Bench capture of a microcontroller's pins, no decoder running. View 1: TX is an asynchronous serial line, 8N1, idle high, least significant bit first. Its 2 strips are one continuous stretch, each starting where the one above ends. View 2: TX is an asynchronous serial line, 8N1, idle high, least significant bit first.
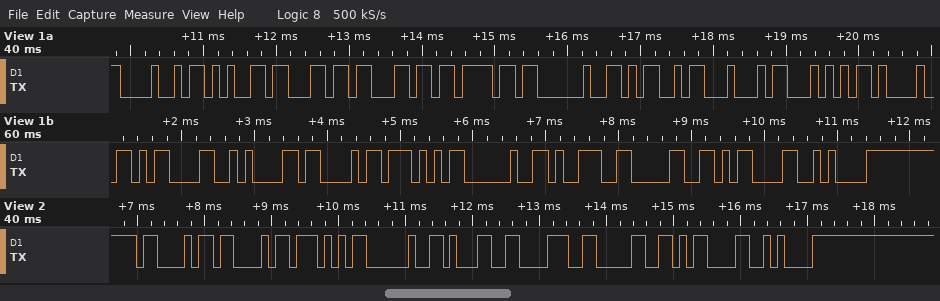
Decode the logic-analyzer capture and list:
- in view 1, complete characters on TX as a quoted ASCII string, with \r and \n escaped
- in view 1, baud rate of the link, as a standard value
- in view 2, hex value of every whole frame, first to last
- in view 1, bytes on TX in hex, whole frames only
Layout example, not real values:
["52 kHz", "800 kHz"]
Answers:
["\"Hello MDT!\\r\\nCW 90\\r\\n\"", "9600 baud", "0x43 0x43 0x57 0x20 0x31 0x38 0x30 0x0D 0x0A", "48 65 6C 6C 6F 20 4D 44 54 21 0D 0A 43 57 20 39 30 0D 0A"]
